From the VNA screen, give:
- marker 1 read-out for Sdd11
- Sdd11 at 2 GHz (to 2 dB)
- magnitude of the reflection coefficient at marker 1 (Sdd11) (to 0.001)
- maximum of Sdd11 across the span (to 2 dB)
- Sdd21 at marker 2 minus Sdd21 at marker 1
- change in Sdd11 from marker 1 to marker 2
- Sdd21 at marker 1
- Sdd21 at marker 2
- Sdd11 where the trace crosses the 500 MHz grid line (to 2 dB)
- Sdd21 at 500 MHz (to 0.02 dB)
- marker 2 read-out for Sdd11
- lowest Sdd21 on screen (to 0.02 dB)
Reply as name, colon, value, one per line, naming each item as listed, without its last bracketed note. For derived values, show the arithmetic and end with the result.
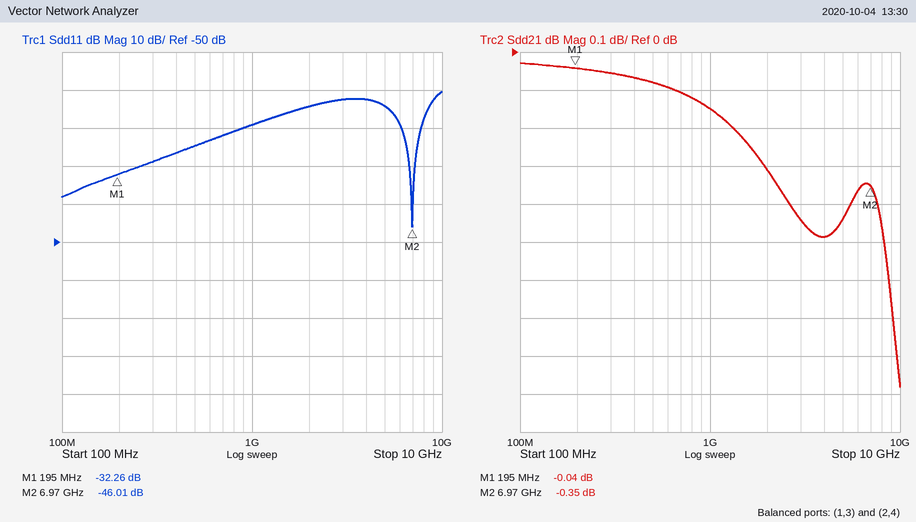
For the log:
marker 1 read-out for Sdd11: -32.26 dB
Sdd11 at 2 GHz: -14 dB
magnitude of the reflection coefficient at marker 1 (Sdd11): 10^(-32.26/20) ≈ 0.024
maximum of Sdd11 across the span: -10 dB
Sdd21 at marker 2 minus Sdd21 at marker 1: -0.35 − (-0.04) = -0.31 dB
change in Sdd11 from marker 1 to marker 2: -46.01 − (-32.26) = -13.75 dB
Sdd21 at marker 1: -0.04 dB
Sdd21 at marker 2: -0.35 dB
Sdd11 where the trace crosses the 500 MHz grid line: -24 dB
Sdd21 at 500 MHz: -0.08 dB
marker 2 read-out for Sdd11: -46.01 dB
lowest Sdd21 on screen: -0.88 dB
